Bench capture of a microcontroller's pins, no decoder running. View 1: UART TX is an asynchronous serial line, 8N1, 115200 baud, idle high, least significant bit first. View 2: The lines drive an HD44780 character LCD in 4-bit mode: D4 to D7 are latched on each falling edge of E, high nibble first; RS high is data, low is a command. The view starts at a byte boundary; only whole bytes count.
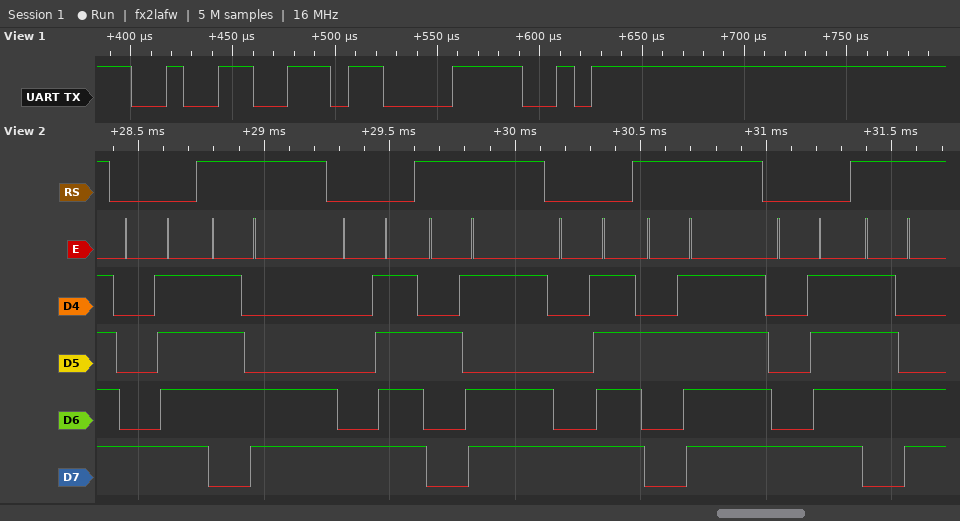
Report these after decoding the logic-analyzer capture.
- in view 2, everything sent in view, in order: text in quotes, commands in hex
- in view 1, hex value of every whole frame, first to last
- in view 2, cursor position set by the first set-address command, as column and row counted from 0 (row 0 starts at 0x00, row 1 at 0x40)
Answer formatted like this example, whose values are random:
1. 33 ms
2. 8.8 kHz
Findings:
1. 0x8F "|" 0x8F "-" 0x8F "/" 0x8F "|"
2. 32 C3 FA
3. column 15, row 0
